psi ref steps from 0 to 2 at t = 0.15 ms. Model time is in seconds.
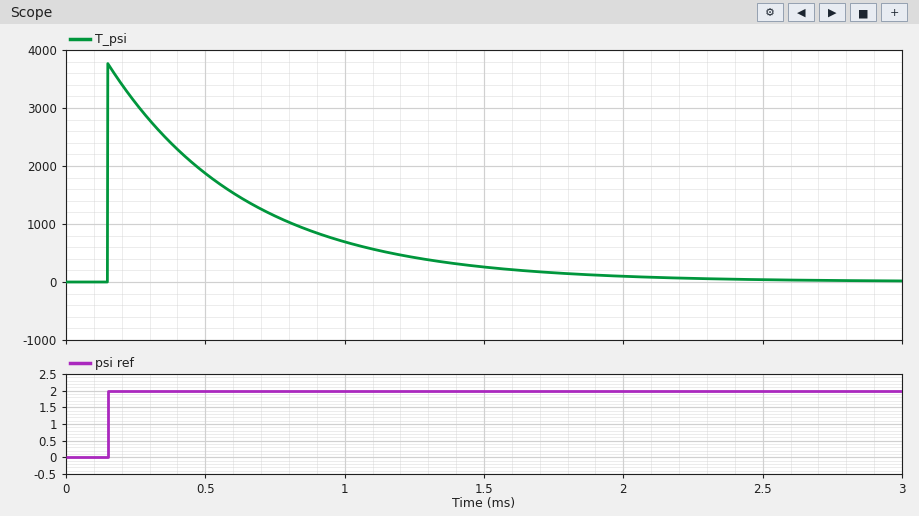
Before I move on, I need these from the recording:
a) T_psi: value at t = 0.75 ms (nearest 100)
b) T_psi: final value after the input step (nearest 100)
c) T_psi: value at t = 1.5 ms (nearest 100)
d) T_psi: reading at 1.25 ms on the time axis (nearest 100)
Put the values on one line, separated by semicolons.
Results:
1100; 0; 300; 400
